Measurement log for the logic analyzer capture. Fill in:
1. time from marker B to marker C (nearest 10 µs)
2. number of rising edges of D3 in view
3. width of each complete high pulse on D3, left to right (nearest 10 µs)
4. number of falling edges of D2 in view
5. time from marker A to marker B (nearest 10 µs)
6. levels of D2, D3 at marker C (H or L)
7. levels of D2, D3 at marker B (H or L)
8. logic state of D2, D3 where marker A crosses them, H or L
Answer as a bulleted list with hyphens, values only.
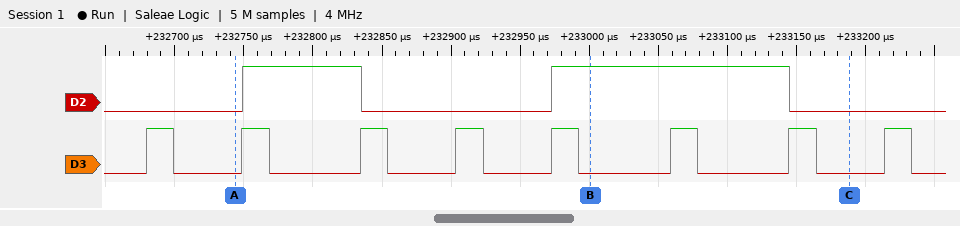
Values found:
- 190 µs
- 8
- 20 µs, 20 µs, 20 µs, 20 µs, 20 µs, 20 µs, 20 µs, 20 µs
- 2
- 260 µs
- D2=L, D3=L
- D2=H, D3=L
- D2=L, D3=L
